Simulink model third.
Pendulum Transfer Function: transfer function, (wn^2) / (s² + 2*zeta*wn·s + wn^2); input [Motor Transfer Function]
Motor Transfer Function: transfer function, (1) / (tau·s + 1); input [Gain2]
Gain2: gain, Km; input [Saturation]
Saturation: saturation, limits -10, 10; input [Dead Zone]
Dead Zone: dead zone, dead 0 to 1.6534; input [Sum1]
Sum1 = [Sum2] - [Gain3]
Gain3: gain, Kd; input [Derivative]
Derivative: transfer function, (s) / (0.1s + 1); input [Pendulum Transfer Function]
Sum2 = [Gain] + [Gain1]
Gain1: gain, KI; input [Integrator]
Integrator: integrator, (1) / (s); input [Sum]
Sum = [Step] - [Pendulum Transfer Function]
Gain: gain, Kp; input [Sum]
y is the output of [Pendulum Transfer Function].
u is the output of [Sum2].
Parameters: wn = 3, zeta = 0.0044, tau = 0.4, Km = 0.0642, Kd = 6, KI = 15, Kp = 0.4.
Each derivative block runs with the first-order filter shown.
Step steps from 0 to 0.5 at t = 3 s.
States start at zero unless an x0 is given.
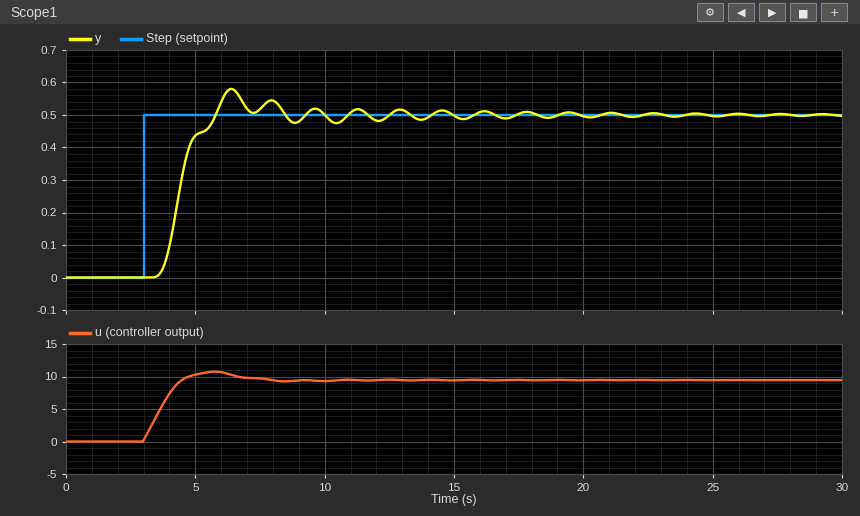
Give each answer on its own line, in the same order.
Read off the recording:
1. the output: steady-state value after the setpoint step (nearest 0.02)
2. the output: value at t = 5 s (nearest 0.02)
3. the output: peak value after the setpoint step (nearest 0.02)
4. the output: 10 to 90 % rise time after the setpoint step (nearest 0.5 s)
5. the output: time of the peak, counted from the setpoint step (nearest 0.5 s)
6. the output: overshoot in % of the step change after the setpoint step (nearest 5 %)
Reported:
0.50
0.44
0.58
1.5 s
3.5 s
15 %
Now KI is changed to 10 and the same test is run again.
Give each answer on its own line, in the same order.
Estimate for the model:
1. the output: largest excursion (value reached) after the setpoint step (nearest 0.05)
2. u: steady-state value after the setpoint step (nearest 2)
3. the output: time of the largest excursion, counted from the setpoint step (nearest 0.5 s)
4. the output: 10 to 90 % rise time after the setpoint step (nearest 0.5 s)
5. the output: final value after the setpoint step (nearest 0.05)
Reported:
0.55
10
5.0 s
2.0 s
0.50
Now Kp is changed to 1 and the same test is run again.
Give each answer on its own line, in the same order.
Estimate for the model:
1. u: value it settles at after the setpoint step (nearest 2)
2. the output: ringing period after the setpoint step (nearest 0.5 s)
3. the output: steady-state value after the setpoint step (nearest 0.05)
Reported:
10
1.5 s
0.50
